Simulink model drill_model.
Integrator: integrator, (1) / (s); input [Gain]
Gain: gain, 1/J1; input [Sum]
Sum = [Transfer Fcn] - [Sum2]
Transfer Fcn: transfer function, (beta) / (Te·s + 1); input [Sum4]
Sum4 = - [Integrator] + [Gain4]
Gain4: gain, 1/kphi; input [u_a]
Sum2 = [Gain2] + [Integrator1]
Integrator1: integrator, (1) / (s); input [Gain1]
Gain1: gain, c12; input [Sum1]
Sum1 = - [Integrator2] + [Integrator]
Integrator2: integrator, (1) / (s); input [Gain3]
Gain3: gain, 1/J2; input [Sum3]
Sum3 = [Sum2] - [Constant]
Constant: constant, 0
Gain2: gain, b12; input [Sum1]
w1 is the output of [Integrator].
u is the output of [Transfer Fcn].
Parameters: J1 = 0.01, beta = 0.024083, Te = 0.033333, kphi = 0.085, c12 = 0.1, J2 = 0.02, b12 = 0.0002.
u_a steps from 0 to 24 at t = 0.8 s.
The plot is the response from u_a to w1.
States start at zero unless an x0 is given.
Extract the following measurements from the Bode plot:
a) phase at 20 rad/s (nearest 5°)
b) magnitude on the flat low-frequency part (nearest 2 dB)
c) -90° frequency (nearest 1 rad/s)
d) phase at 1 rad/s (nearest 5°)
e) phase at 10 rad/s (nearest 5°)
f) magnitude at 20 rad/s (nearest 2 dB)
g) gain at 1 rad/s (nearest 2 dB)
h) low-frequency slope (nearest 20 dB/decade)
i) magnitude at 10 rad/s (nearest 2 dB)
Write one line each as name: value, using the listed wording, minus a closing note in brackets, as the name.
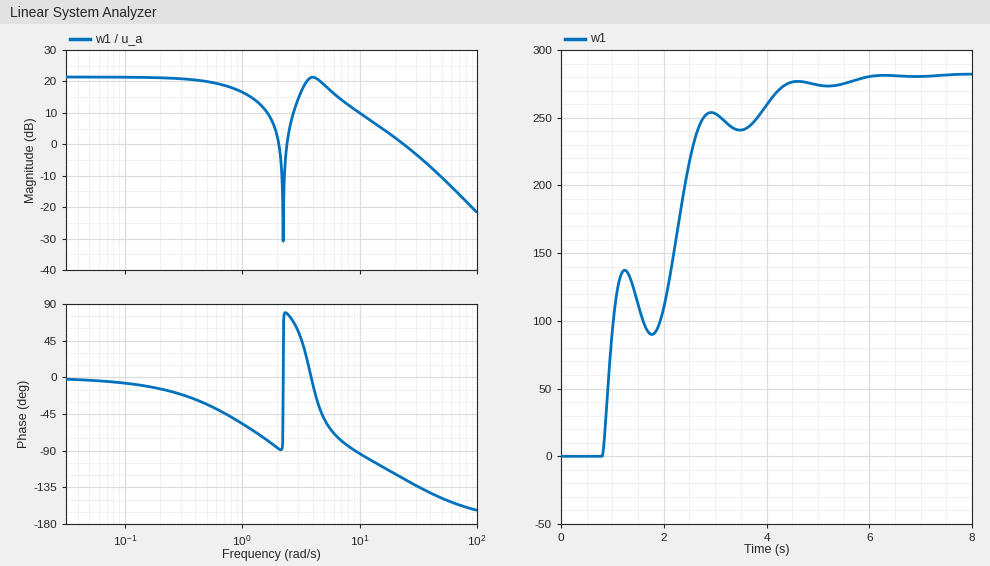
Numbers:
phase at 20 rad/s: -120°
magnitude on the flat low-frequency part: 22 dB
-90° frequency: 9 rad/s
phase at 1 rad/s: -55°
phase at 10 rad/s: -95°
magnitude at 20 rad/s: 2 dB
gain at 1 rad/s: 16 dB
low-frequency slope: 0 dB/decade
magnitude at 10 rad/s: 10 dB
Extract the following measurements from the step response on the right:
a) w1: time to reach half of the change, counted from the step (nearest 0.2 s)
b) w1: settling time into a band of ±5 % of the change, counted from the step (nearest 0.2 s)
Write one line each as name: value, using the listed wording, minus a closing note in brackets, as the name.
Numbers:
w1: time to reach half of the change, counted from the step: 1.4 s
w1: settling time into a band of ±5 % of the change, counted from the step: 3.4 s
